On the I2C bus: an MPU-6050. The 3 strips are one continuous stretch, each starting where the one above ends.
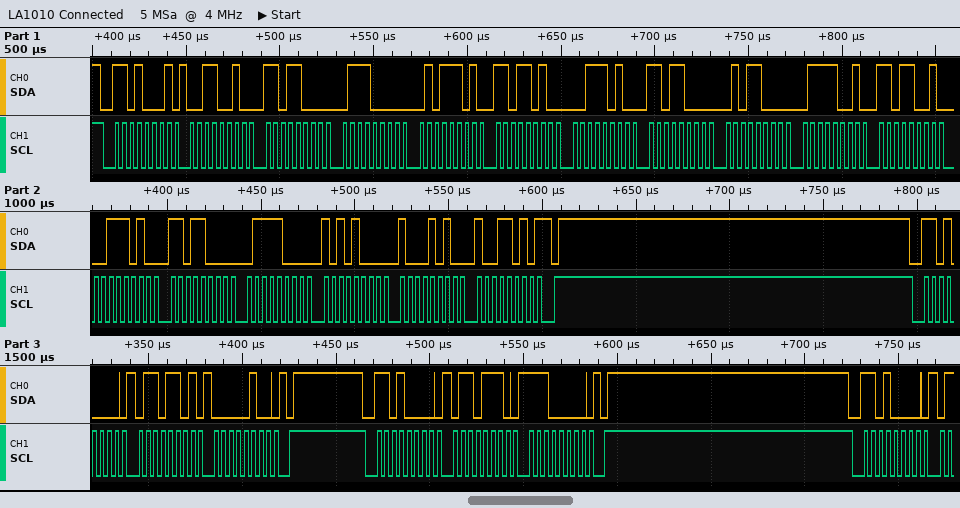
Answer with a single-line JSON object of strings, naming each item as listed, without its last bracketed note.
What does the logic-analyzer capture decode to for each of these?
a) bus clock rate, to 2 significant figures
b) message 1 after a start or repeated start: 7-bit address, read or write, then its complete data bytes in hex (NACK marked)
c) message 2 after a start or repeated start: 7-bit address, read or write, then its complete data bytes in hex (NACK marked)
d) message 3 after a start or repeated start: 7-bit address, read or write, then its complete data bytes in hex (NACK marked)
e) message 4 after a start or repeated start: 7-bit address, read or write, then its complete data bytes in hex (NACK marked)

{"bus clock rate, to 2 significant figures": "250 kHz", "message 1 after a start or repeated start: 7-bit address, read or write, then its complete data bytes in hex": "0x68 read: 32 D8 70 5D DA 3A D8 58 79 D9 3A D8 78 A8 8A 9A NACK", "message 2 after a start or repeated start: 7-bit address, read or write, then its complete data bytes in hex": "0x68 write: 6D 04", "message 3 after a start or repeated start: 7-bit address, read or write, then its complete data bytes in hex": "0x68 write: 6E E0", "message 4 after a start or repeated start: 7-bit address, read or write, then its complete data bytes in hex": "0x68 write"}
